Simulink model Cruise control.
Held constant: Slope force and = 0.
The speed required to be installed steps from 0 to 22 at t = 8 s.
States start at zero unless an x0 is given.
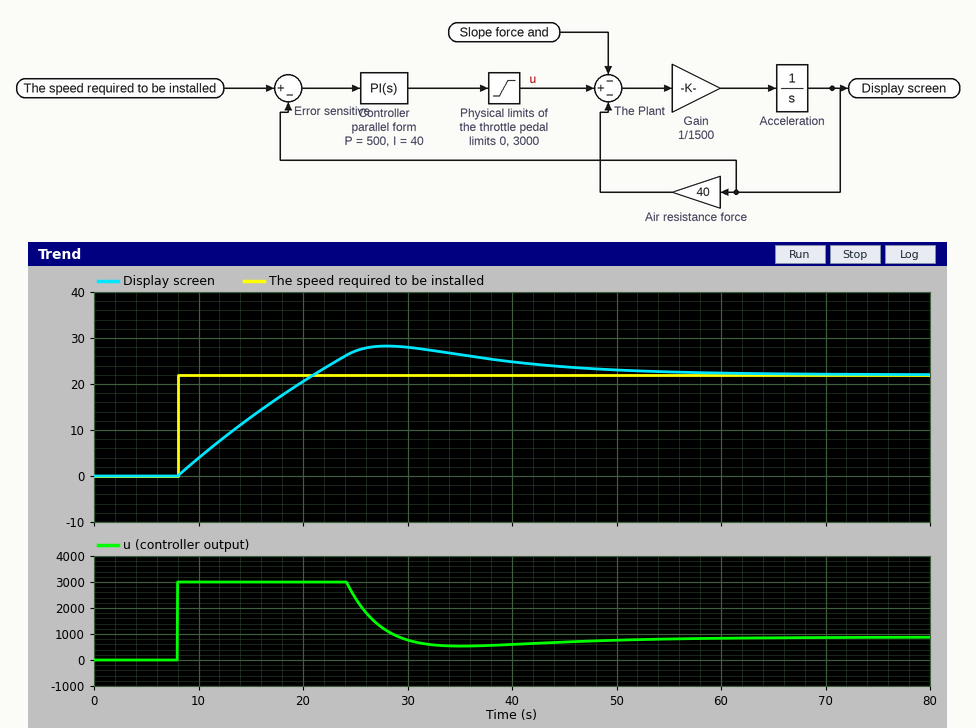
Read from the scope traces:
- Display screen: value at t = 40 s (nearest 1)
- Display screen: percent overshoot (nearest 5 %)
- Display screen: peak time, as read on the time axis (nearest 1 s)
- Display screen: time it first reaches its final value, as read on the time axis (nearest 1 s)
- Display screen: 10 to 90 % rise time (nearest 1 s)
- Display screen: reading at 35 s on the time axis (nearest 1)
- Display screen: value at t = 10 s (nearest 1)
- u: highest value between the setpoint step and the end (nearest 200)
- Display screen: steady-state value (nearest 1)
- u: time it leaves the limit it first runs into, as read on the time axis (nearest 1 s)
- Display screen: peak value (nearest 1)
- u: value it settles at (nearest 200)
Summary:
25
30 %
28 s
21 s
10 s
26
4
3000
22
24 s
28
800
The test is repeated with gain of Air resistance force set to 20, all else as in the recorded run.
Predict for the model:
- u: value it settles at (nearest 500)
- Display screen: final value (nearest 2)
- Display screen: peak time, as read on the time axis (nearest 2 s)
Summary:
500
22
26 s
